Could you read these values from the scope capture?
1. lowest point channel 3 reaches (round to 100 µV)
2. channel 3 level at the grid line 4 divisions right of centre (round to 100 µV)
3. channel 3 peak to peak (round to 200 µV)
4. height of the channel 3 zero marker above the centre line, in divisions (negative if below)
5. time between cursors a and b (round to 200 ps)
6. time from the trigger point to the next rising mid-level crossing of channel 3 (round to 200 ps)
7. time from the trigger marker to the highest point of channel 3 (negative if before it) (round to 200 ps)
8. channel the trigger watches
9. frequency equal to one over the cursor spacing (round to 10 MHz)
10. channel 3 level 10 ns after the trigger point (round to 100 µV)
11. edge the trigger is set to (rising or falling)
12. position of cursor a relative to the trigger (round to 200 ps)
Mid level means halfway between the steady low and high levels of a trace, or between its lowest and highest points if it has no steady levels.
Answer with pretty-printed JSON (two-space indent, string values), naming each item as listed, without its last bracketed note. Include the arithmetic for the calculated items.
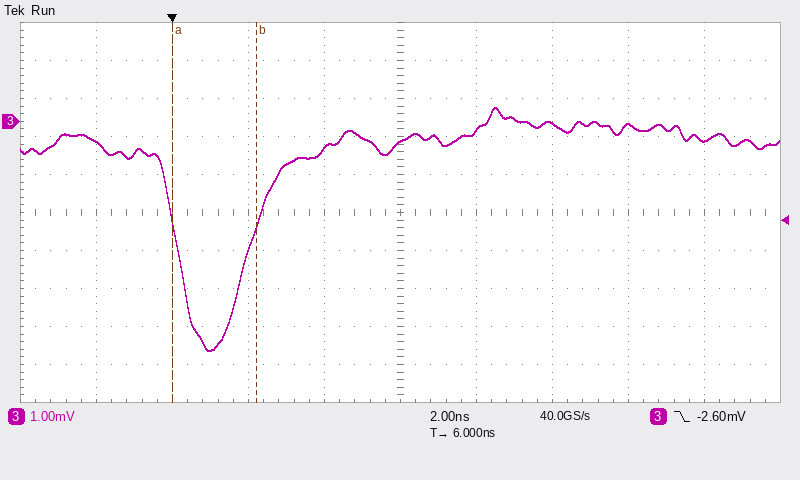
{
  "lowest point channel 3 reaches": "-6.0 mV",
  "channel 3 level at the grid line 4 divisions right of centre": "-500 µV",
  "channel 3 peak to peak": "6.4 mV",
  "height of the channel 3 zero marker above the centre line, in divisions": "+2.4 div",
  "time between cursors a and b": "2.2 ns",
  "time from the trigger point to the next rising mid-level crossing of channel 3": "2.2 ns",
  "time from the trigger marker to the highest point of channel 3 (negative if before it)": "+8.6 ns",
  "channel the trigger watches": "channel 3",
  "frequency equal to one over the cursor spacing": "1 / 2.2 ns ≈ 450 MHz",
  "channel 3 level 10 ns after the trigger point": "-100 µV",
  "edge the trigger is set to": "falling",
  "position of cursor a relative to the trigger": "0.0 ns"
}
